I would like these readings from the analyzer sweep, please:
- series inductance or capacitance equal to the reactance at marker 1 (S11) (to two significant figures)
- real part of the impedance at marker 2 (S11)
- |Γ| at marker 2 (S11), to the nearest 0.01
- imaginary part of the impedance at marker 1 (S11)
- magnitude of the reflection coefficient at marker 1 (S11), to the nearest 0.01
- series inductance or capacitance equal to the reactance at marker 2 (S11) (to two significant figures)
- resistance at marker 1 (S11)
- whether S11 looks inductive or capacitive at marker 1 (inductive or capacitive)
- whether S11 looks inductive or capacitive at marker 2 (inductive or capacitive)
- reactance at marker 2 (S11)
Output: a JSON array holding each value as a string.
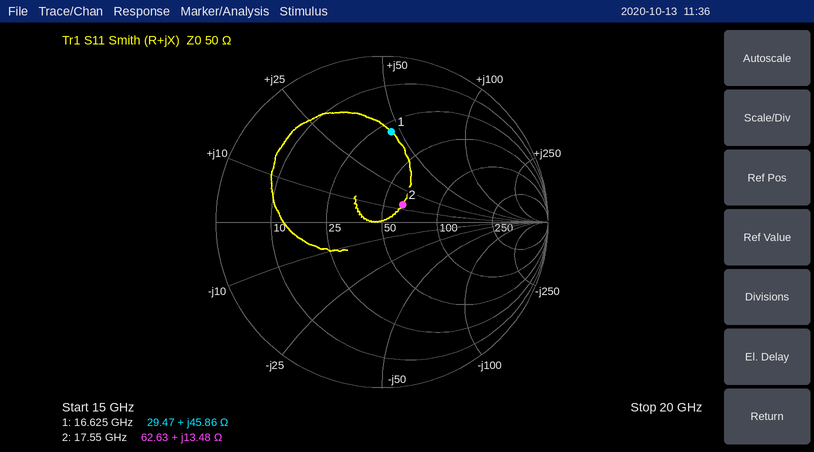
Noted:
["440 pH", "62.63 Ω", "0.16", "+45.86 Ω", "0.55", "120 pH", "29.47 Ω", "inductive", "inductive", "+13.48 Ω"]
